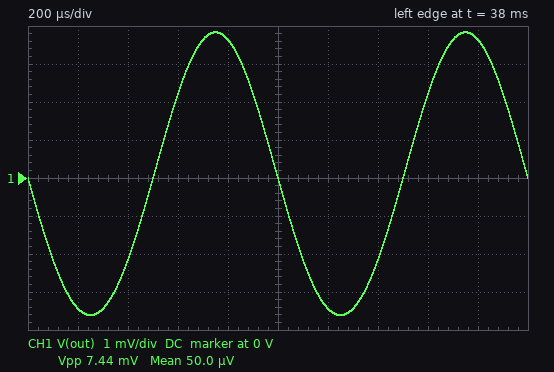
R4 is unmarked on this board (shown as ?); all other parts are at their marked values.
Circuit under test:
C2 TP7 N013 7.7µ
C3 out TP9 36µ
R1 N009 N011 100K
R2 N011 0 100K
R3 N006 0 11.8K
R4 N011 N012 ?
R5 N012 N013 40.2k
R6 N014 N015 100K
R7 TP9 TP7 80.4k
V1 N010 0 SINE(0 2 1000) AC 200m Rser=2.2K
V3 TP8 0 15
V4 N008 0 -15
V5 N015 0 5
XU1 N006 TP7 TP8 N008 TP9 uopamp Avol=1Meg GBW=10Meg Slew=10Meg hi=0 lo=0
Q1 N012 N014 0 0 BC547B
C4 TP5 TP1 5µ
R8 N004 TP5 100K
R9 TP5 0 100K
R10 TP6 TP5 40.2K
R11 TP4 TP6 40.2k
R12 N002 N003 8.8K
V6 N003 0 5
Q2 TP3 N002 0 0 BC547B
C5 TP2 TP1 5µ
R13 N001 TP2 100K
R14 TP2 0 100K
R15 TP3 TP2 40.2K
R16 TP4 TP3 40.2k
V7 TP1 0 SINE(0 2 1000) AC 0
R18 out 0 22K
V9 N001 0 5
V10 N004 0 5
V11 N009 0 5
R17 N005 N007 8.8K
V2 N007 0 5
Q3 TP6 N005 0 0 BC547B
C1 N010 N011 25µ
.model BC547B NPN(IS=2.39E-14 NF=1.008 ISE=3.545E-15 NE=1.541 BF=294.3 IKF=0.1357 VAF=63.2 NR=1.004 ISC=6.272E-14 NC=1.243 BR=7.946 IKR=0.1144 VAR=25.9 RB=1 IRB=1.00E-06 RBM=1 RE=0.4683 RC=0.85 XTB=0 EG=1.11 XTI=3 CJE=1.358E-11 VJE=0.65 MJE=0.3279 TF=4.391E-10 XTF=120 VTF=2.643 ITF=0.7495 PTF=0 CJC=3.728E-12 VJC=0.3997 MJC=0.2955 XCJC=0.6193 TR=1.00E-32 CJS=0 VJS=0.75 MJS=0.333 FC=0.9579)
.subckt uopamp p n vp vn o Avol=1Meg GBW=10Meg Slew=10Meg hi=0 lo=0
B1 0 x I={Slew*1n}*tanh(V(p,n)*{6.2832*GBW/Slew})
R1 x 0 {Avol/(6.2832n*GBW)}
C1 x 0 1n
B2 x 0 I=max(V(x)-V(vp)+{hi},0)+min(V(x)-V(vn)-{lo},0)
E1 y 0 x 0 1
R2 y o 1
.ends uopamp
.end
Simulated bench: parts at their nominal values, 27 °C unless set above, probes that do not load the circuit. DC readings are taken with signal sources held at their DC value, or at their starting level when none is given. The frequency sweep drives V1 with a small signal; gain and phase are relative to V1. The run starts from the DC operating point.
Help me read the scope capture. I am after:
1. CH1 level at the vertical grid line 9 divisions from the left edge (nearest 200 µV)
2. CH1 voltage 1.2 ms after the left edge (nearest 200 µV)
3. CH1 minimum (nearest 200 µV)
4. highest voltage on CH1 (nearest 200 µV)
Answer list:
3.6 mV
-3.4 mV
-3.6 mV
3.8 mV
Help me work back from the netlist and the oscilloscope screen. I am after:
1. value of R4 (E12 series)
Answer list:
82 kΩ
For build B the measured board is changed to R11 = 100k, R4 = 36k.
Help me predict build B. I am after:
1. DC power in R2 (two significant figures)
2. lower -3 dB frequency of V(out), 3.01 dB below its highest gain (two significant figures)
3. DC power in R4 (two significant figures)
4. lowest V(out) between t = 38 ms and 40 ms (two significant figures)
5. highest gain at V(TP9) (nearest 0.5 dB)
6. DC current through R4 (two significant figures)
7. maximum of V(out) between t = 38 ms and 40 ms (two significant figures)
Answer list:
11 µW
680 mHz
30 µW
-7.5 mV
-48.0 dB
29 µA
8.5 mV
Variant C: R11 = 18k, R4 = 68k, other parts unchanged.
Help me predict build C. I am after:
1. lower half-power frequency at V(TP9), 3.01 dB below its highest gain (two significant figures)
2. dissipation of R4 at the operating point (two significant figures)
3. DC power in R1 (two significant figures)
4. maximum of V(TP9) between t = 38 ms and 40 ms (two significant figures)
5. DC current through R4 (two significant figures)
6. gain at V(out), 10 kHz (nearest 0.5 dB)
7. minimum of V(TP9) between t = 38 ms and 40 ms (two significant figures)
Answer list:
580 mHz
30 µW
130 µW
4.6 mV
21 µA
-53.0 dB
-4.3 mV
